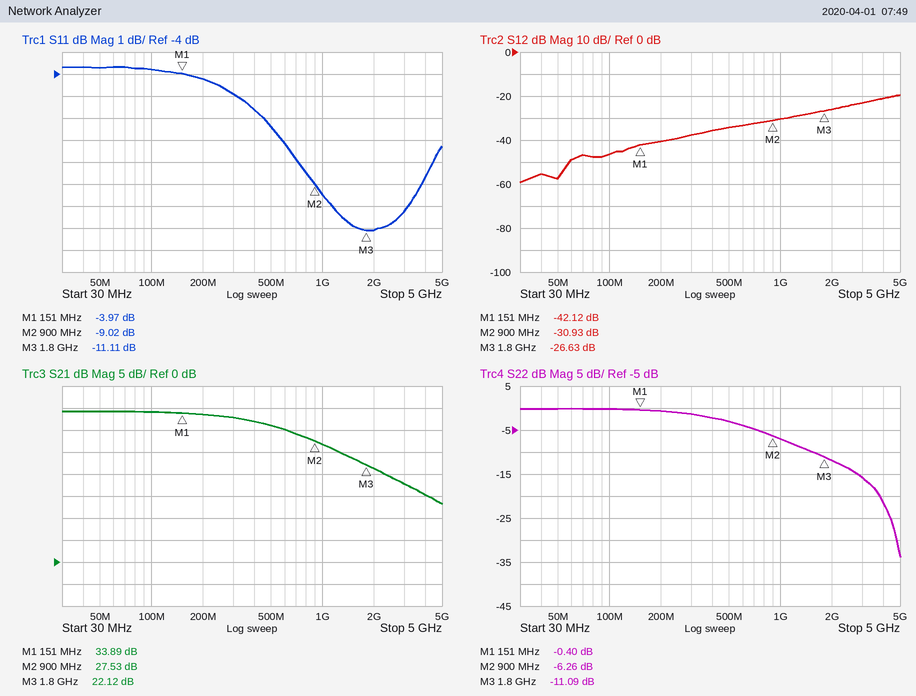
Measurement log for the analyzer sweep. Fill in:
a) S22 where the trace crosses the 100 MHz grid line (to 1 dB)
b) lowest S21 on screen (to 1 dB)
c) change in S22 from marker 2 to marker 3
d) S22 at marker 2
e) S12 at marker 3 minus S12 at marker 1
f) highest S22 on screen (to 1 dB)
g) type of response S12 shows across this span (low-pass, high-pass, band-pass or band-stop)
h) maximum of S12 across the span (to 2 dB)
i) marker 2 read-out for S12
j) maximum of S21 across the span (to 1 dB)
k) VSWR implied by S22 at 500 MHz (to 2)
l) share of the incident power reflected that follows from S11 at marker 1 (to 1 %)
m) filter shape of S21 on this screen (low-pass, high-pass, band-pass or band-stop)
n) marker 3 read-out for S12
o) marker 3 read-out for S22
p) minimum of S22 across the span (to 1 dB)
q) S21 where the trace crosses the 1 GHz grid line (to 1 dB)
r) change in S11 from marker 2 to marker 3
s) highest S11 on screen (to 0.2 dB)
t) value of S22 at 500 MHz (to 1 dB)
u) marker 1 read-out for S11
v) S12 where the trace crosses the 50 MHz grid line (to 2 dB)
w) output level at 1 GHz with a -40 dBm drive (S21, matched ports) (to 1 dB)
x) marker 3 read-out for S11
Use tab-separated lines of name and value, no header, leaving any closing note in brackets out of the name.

S22 where the trace crosses the 100 MHz grid line	0 dB
lowest S21 on screen	13 dB
change in S22 from marker 2 to marker 3	-4.83 dB
S22 at marker 2	-6.26 dB
S12 at marker 3 minus S12 at marker 1	15.49 dB
highest S22 on screen	0 dB
type of response S12 shows across this span	high-pass
maximum of S12 across the span	-20 dB
marker 2 read-out for S12	-30.93 dB
maximum of S21 across the span	34 dB
VSWR implied by S22 at 500 MHz	6
share of the incident power reflected that follows from S11 at marker 1	40 %
filter shape of S21 on this screen	low-pass
marker 3 read-out for S12	-26.63 dB
marker 3 read-out for S22	-11.09 dB
minimum of S22 across the span	-34 dB
S21 where the trace crosses the 1 GHz grid line	27 dB
change in S11 from marker 2 to marker 3	-2.09 dB
highest S11 on screen	-3.6 dB
value of S22 at 500 MHz	-3 dB
marker 1 read-out for S11	-3.97 dB
S12 where the trace crosses the 50 MHz grid line	-58 dB
output level at 1 GHz with a -40 dBm drive (S21, matched ports)	-13 dBm
marker 3 read-out for S11	-11.11 dB
